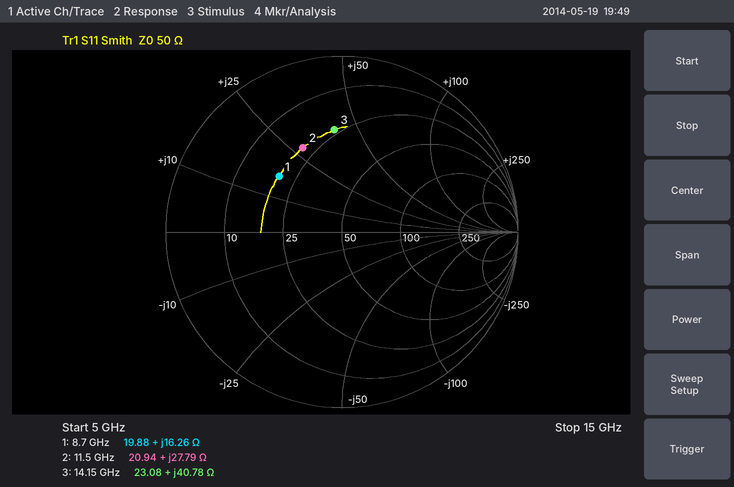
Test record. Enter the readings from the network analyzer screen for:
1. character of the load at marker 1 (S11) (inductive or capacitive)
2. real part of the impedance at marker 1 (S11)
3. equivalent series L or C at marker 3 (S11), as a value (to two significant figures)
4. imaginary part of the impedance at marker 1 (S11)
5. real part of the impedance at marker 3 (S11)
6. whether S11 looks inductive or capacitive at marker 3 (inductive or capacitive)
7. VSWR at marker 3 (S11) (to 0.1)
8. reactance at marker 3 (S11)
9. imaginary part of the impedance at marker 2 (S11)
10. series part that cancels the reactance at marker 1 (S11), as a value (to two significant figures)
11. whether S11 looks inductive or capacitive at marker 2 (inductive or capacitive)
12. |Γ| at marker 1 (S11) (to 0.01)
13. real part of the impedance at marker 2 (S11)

inductive
19.88 Ω
460 pH
+16.26 Ω
23.08 Ω
inductive
3.8
+40.78 Ω
+27.79 Ω
1.1 pF
inductive
0.48
20.94 Ω
